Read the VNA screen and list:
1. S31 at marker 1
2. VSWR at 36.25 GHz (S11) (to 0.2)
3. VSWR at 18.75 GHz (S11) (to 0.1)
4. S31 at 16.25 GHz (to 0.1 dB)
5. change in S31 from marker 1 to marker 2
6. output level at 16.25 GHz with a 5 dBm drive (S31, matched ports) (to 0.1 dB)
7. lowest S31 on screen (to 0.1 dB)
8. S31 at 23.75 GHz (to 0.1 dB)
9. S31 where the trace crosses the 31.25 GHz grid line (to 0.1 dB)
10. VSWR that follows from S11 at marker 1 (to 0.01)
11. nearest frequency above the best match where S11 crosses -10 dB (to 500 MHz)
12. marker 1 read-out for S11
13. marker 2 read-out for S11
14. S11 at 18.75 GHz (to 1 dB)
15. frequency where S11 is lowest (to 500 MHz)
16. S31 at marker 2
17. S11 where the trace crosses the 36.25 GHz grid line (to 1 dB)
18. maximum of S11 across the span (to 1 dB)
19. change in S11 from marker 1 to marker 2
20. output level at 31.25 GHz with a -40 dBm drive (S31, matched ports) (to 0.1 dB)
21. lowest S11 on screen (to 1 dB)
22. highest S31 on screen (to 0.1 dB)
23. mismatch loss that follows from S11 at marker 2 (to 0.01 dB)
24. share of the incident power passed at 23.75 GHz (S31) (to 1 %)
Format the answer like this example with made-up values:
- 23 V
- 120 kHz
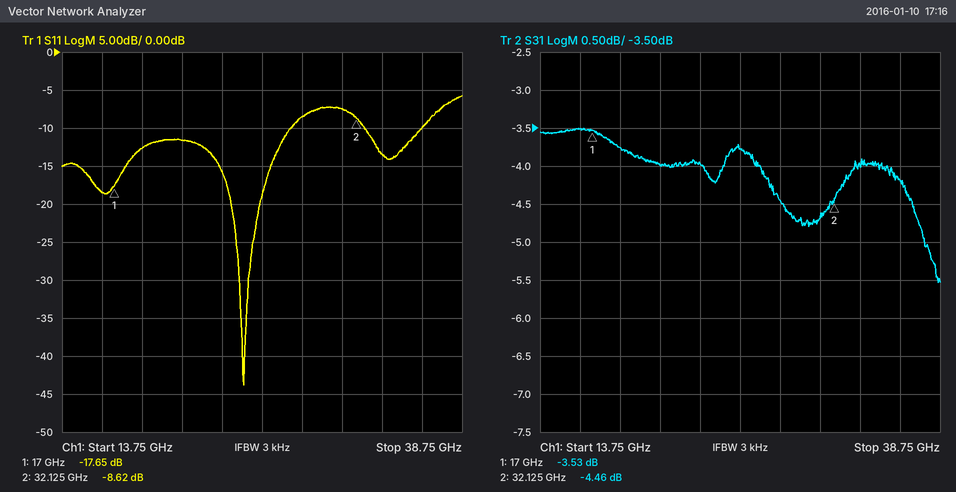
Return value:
- -3.53 dB
- 2.0
- 1.6
- -3.5 dB
- -0.93 dB
- 1.5 dBm
- -5.5 dB
- -4.0 dB
- -4.7 dB
- 1.30
- 28.0 GHz
- -17.65 dB
- -8.62 dB
- -13 dB
- 25.0 GHz
- -4.46 dB
- -10 dB
- -6 dB
- 9.03 dB
- -44.7 dBm
- -44 dB
- -3.5 dB
- 0.64 dB
- 40 %
